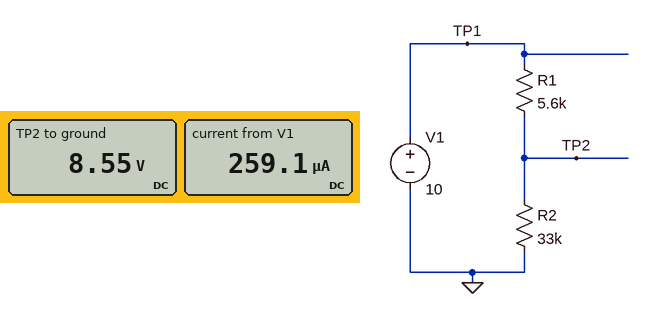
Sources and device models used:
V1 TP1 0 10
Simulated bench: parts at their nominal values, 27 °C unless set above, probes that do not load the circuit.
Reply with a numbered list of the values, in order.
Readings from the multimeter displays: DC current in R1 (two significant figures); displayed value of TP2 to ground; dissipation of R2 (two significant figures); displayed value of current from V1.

1. 260 µA
2. 8.55 V
3. 2.2 mW
4. 259.1 µA
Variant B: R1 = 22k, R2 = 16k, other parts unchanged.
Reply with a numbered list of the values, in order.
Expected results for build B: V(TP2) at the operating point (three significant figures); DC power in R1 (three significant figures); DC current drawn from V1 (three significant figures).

1. 4.21 V
2. 1.52 mW
3. 263 µA
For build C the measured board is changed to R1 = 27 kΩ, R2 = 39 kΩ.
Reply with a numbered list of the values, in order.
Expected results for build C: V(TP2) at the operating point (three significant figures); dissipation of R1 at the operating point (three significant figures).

1. 5.91 V
2. 620 µW
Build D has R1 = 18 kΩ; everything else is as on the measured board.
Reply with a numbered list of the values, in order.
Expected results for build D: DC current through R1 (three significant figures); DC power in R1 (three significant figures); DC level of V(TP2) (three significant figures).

1. 196 µA
2. 692 µW
3. 6.47 V
